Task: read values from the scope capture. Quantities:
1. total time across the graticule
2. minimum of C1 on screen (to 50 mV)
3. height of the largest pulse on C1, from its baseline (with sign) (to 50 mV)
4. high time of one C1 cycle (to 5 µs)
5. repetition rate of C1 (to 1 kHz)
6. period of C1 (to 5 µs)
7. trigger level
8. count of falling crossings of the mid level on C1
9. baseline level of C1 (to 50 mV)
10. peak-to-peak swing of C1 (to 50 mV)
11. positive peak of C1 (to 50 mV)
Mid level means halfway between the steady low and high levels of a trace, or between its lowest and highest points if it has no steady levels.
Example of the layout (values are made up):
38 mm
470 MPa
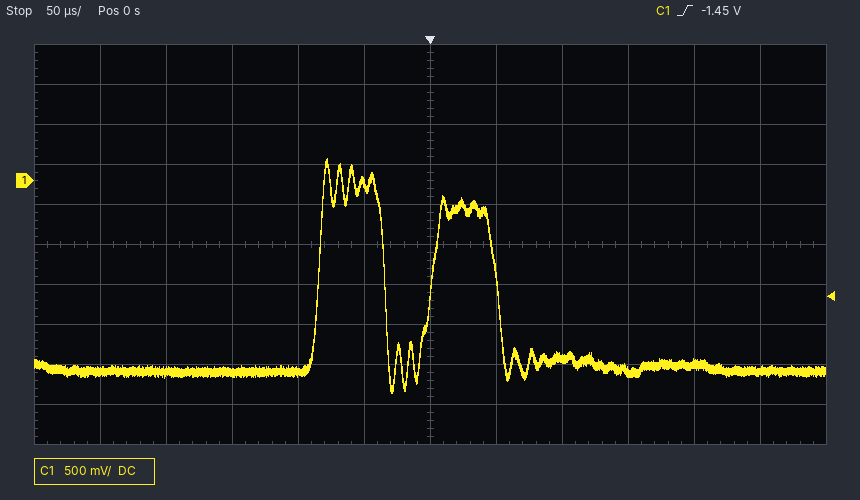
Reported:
600 µs
-2.65 V
+2.65 V
50 µs
12 kHz
85 µs
-1.45 V
2
-2.40 V
2.90 V
250 mV
